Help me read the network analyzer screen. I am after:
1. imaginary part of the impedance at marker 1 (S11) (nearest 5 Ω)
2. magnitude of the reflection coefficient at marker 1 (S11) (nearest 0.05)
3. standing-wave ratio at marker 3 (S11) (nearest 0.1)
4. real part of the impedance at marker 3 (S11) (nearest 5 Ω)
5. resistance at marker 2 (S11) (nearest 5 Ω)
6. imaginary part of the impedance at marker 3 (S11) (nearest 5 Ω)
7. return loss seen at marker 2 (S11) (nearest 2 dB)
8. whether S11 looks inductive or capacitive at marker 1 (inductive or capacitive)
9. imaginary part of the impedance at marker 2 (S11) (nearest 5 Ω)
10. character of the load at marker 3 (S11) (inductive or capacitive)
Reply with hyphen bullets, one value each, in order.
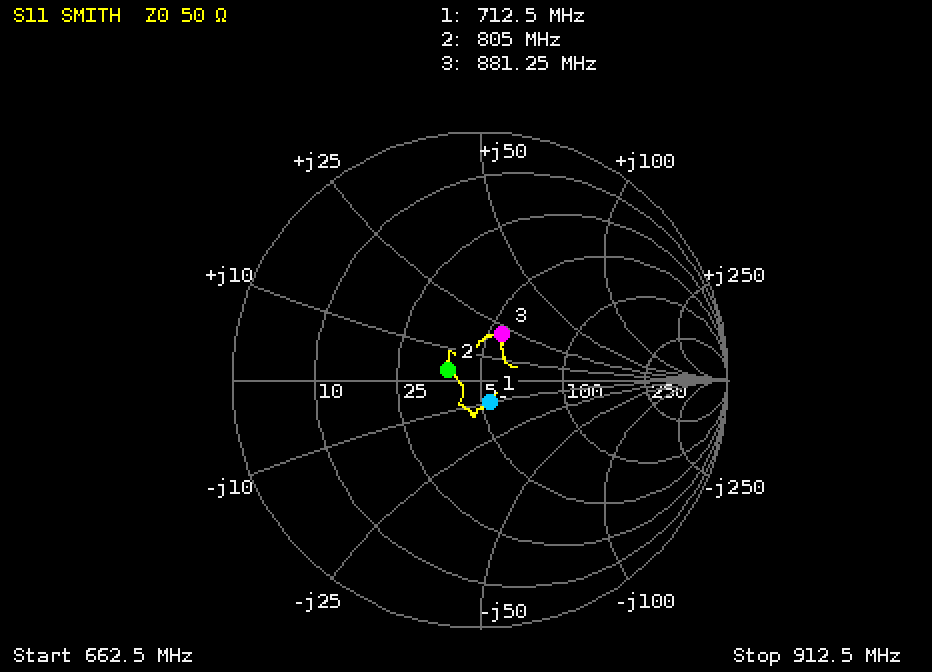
- -10 Ω
- 0.10
- 1.5
- 55 Ω
- 40 Ω
- +20 Ω
- 18 dB
- capacitive
- +5 Ω
- inductive
